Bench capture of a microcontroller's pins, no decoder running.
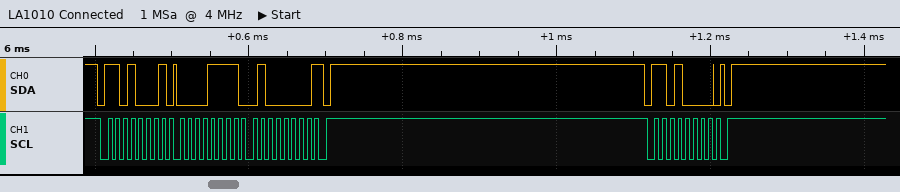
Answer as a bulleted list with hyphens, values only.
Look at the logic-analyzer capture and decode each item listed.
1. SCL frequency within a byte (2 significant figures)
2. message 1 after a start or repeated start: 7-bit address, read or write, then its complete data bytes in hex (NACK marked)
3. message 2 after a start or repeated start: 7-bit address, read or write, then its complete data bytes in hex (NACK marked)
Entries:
- 100 kHz
- 0x68 read: 0F 40 NACK
- 0x68 write
